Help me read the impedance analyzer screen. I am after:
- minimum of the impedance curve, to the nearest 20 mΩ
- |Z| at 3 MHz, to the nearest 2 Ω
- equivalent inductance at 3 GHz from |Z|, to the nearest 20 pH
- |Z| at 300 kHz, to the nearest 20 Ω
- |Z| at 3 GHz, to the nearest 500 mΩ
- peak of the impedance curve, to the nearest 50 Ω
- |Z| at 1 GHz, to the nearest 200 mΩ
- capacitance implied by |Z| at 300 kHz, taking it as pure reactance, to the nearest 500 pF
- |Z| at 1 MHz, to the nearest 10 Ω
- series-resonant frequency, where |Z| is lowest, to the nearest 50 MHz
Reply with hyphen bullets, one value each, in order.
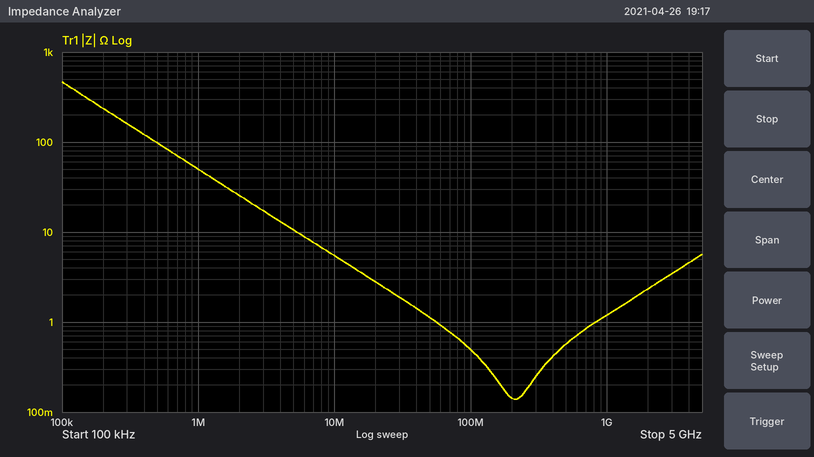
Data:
- 140 mΩ
- 18 Ω
- 180 pH
- 160 Ω
- 3.5 Ω
- 450 Ω
- 1.2 Ω
- 3.5 nF
- 50 Ω
- 200 MHz
